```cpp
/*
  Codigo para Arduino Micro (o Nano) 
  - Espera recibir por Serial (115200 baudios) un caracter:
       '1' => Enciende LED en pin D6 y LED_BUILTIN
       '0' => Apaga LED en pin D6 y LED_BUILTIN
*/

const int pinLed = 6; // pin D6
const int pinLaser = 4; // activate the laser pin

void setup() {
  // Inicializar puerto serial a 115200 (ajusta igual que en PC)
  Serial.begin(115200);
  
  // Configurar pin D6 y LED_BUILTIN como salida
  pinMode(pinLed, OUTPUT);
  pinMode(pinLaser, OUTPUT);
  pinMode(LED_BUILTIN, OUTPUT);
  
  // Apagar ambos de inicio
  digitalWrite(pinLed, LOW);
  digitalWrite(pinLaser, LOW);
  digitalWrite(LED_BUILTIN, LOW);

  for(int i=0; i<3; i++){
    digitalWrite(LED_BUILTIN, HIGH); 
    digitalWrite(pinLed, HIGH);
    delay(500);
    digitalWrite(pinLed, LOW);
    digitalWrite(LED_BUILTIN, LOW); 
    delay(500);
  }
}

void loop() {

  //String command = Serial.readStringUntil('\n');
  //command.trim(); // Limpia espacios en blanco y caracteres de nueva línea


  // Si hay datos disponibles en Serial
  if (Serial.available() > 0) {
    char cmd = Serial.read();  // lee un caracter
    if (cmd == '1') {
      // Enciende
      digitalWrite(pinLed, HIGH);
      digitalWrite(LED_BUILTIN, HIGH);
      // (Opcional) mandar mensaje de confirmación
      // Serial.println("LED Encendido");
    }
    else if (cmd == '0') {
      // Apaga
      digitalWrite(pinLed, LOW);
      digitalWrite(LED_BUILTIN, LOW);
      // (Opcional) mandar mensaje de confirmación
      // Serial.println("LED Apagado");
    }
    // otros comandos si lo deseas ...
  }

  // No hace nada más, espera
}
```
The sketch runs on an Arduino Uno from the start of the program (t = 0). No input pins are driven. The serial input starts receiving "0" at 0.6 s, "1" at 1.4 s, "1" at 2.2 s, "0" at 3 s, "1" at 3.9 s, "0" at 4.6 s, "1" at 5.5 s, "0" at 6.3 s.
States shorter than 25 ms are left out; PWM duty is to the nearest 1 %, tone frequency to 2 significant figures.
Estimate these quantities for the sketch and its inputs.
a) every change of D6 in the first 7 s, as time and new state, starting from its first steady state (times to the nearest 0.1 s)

0 s high; 0.5 s low; 1 s high; 1.5 s low; 2 s high; 2.5 s low; 3.9 s high; 4.6 s low; 5.5 s high; 6.3 s low
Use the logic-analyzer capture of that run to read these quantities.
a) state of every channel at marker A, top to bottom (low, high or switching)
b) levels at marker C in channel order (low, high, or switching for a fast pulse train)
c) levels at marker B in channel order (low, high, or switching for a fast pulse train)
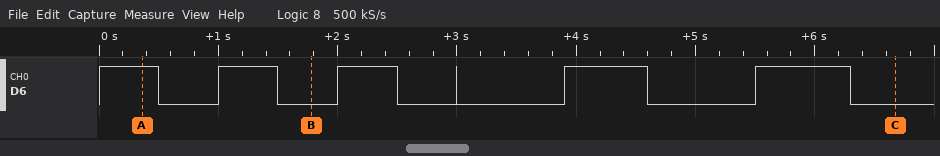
D6 high
D6 low
D6 low
